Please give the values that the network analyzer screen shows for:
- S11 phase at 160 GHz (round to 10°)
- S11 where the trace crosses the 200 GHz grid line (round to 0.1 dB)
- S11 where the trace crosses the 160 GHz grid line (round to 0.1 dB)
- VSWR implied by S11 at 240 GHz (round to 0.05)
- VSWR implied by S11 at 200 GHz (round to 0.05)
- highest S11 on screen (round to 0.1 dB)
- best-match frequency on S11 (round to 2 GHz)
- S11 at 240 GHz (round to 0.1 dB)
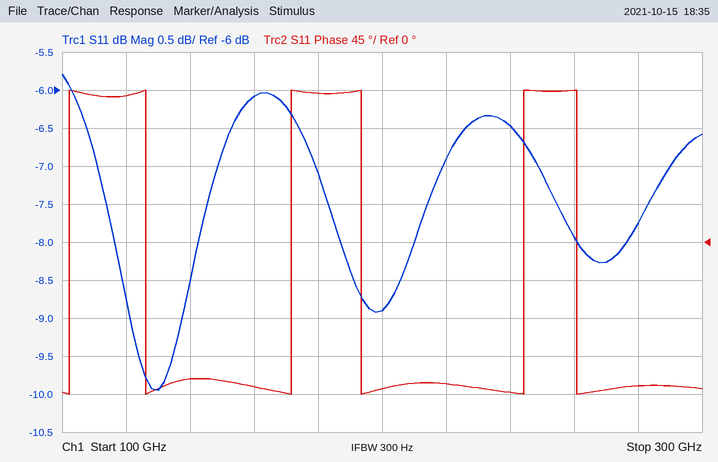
-170°
-8.9 dB
-6.1 dB
2.80
2.10
-5.8 dB
130 GHz
-6.5 dB
